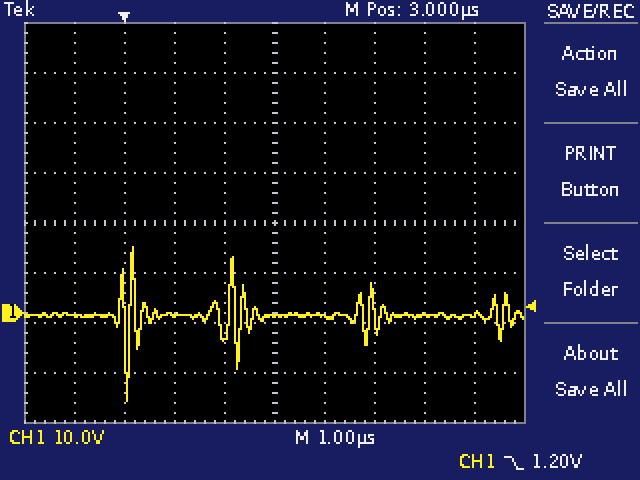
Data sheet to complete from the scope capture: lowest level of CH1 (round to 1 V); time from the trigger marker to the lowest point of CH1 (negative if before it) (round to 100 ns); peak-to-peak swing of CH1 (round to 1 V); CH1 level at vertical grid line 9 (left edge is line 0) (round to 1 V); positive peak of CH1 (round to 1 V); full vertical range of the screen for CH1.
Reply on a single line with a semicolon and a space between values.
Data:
-18 V; +100 ns; 31 V; 0 V; 13 V; 80 V
